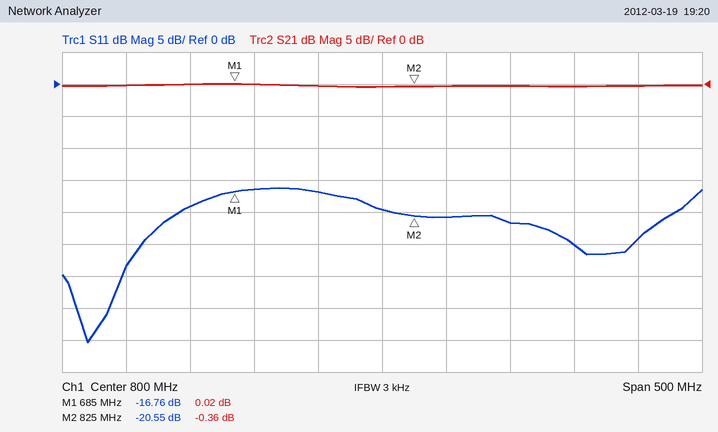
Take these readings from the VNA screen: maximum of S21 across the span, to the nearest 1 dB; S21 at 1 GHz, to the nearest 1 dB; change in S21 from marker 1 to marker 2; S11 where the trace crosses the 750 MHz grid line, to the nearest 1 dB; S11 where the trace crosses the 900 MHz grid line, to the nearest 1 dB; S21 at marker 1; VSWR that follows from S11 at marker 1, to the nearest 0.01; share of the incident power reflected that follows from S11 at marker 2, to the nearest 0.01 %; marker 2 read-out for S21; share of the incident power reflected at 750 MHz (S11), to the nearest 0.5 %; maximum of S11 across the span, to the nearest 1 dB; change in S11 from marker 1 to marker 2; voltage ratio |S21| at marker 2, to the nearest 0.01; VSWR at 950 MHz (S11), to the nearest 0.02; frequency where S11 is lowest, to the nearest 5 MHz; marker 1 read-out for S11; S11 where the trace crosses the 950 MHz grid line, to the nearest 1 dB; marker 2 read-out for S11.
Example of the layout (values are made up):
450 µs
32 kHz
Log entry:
0 dB
0 dB
-0.38 dB
-17 dB
-22 dB
0.02 dB
1.34
0.88 %
-0.36 dB
2.0 %
-16 dB
-3.79 dB
0.96
1.12
570 MHz
-16.76 dB
-25 dB
-20.55 dB
